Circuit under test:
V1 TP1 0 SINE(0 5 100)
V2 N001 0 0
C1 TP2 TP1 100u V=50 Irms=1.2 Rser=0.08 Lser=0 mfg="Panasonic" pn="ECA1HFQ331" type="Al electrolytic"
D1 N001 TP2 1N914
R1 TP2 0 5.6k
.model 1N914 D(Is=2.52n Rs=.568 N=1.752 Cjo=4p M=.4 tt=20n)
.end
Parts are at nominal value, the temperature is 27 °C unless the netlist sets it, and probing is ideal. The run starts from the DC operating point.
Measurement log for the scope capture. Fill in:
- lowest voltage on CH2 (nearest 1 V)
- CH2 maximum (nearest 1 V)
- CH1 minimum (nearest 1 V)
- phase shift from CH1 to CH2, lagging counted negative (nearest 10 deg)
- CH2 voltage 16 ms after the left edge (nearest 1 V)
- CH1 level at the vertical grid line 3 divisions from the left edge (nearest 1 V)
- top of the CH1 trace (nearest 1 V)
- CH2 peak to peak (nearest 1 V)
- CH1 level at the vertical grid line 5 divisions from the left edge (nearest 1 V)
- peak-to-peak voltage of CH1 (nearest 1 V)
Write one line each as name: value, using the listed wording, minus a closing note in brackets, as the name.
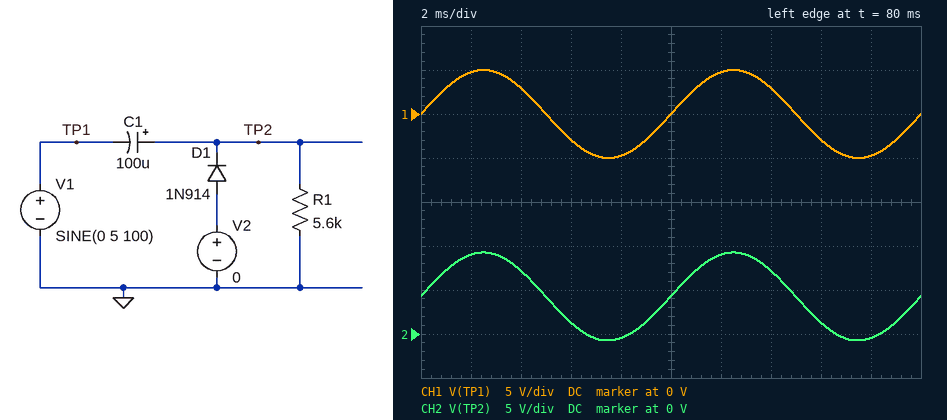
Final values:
lowest voltage on CH2: -1 V
CH2 maximum: 9 V
CH1 minimum: -5 V
phase shift from CH1 to CH2, lagging counted negative: 0 deg
CH2 voltage 16 ms after the left edge: 1 V
CH1 level at the vertical grid line 3 divisions from the left edge: -3 V
top of the CH1 trace: 5 V
CH2 peak to peak: 10 V
CH1 level at the vertical grid line 5 divisions from the left edge: 0 V
peak-to-peak voltage of CH1: 10 V
